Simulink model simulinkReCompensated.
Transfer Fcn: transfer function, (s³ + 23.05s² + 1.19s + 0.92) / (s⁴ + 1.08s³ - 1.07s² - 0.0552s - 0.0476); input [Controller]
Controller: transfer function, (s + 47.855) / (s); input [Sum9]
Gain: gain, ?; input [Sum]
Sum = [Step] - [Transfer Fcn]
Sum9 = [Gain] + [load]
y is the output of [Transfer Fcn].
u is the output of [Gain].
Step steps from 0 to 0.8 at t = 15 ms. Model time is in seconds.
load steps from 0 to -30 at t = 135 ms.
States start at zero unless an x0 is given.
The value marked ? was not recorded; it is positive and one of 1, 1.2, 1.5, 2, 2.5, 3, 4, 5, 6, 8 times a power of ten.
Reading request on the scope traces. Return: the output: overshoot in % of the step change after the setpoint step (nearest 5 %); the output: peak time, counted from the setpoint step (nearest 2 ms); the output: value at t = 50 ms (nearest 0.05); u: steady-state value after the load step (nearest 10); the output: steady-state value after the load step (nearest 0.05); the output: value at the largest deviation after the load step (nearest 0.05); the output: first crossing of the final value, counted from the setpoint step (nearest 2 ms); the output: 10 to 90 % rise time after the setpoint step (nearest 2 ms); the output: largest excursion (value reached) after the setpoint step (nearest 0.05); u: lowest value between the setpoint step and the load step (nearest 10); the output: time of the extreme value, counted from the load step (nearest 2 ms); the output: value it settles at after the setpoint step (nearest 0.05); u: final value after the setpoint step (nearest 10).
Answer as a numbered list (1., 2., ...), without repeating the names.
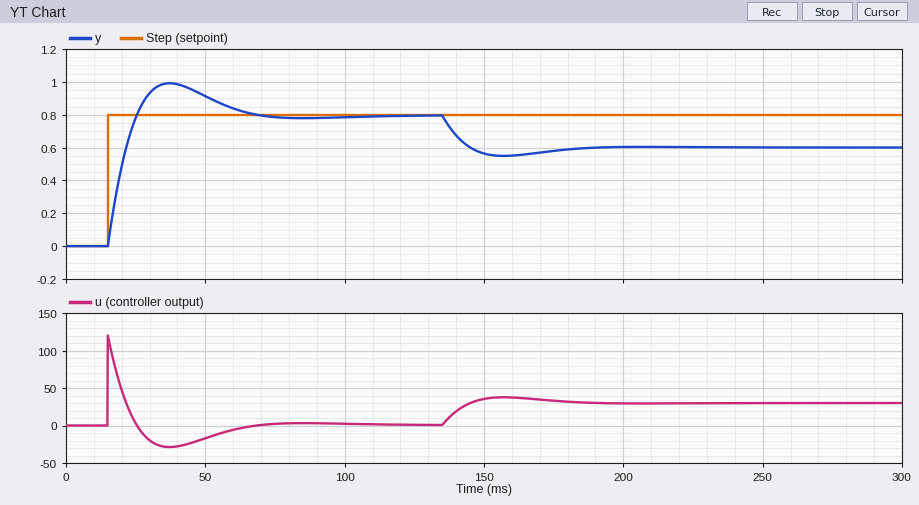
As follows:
1. 25 %
2. 22 ms
3. 0.90
4. 30
5. 0.60
6. 0.55
7. 10 ms
8. 8 ms
9. 1.00
10. -30
11. 22 ms
12. 0.80
13. 0
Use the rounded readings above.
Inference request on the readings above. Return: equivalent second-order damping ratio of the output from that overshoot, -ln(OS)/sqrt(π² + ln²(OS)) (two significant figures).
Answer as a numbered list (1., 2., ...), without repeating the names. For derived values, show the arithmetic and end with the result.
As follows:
1. ln(0.25) = -1.386; 1.386 / sqrt(9.870 + 1.922) = 0.40
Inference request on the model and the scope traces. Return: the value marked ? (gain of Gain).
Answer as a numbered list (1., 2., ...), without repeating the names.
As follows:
1. 150
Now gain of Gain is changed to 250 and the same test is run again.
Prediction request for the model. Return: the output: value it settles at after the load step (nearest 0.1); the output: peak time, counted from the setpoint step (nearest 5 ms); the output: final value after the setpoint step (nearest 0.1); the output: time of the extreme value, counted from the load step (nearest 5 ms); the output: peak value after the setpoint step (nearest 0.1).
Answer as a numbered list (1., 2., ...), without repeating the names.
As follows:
1. 0.7
2. 15 ms
3. 0.8
4. 15 ms
5. 0.9
